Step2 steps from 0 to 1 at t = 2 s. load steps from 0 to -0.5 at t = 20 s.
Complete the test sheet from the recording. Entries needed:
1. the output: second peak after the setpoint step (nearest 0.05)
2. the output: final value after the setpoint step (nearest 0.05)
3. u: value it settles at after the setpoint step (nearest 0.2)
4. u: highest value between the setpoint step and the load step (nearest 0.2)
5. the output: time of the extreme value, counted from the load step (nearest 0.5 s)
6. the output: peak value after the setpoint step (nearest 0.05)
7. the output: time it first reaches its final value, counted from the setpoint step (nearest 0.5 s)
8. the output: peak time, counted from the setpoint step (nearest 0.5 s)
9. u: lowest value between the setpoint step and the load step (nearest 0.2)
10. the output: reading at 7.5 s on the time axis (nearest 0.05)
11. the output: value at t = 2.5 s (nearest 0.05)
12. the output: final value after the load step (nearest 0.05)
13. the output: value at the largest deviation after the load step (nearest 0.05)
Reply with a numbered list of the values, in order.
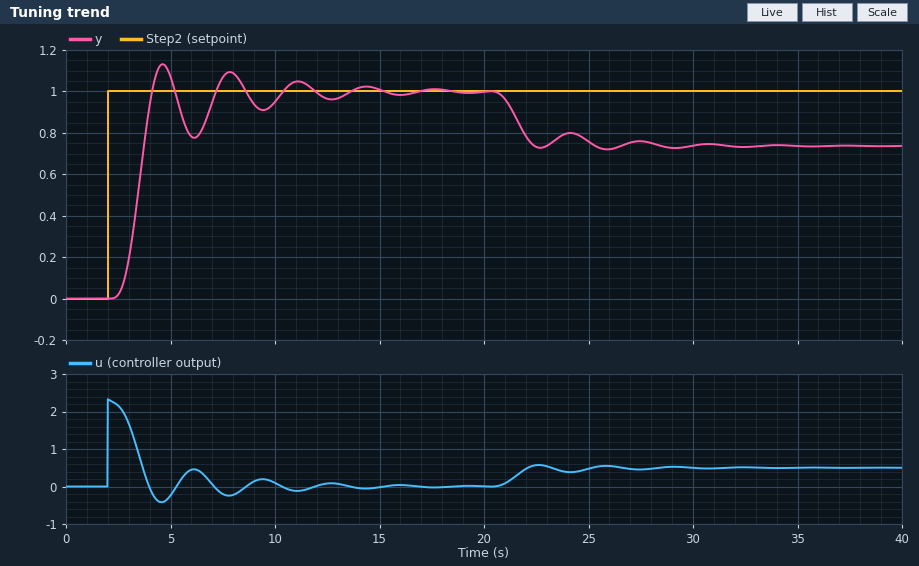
1. 1.10
2. 1.00
3. 0.0
4. 2.4
5. 6.0 s
6. 1.15
7. 2.0 s
8. 2.5 s
9. -0.4
10. 1.05
11. 0.00
12. 0.75
13. 0.70
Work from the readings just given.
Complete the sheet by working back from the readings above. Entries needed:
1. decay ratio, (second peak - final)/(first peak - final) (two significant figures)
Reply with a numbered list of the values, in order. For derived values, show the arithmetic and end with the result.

1. (1.1 - 1) / (1.15 - 1) = 0.67
